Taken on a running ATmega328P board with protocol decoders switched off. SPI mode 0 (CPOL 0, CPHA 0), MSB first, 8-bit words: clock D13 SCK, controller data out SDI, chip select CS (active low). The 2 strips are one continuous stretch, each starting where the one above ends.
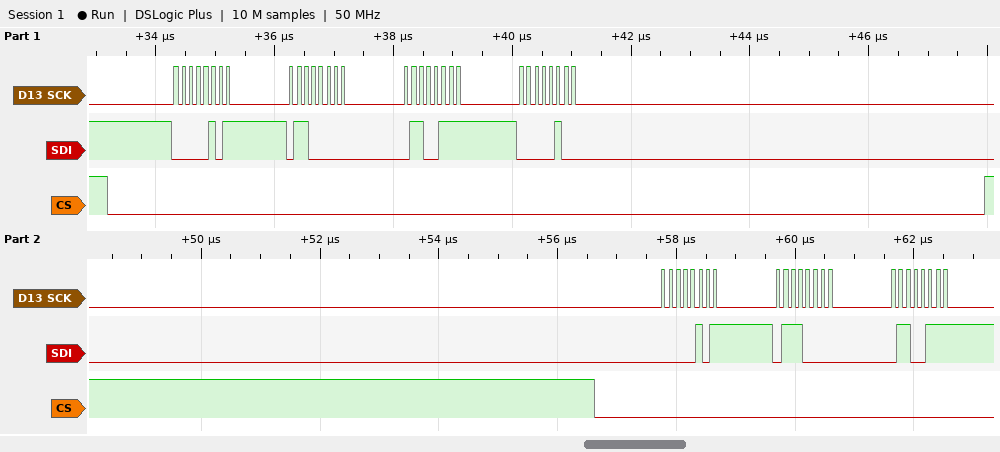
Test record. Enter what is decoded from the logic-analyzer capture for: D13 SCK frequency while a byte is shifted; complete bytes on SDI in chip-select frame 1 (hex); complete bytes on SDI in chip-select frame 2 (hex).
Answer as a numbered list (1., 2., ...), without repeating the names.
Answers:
1. 8 MHz
2. 05 60 67 04
3. 05 70 67
